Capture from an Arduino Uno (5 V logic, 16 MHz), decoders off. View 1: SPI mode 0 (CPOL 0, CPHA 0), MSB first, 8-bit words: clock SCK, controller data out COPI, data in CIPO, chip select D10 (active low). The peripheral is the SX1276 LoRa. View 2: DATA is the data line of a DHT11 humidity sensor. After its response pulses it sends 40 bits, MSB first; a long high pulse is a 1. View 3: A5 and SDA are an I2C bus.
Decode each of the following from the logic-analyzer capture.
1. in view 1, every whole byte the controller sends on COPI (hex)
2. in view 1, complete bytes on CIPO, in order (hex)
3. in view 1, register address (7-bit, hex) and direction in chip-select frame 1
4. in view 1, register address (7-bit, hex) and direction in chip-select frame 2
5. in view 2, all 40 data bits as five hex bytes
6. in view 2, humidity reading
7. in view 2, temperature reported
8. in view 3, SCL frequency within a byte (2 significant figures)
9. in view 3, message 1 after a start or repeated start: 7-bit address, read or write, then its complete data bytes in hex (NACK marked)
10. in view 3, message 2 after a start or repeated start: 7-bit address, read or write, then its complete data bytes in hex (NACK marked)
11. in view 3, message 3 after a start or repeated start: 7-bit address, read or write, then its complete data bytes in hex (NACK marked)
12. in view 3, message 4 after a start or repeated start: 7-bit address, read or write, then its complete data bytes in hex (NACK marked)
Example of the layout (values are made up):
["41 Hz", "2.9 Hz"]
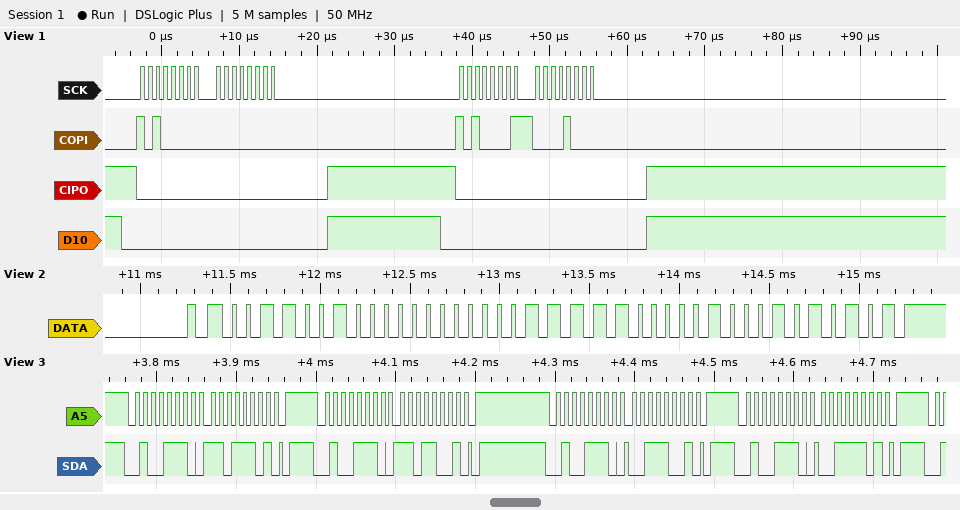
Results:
["A0 00 A1 08", "00 00 00 00", "0x20 write", "0x21 write", "32 00 1F 04 55", "50 %", "31.4 °C", "100 kHz", "0x27 write: DD", "0x27 write: D9", "0x27 write: 39", "0x27 write: 3D"]
